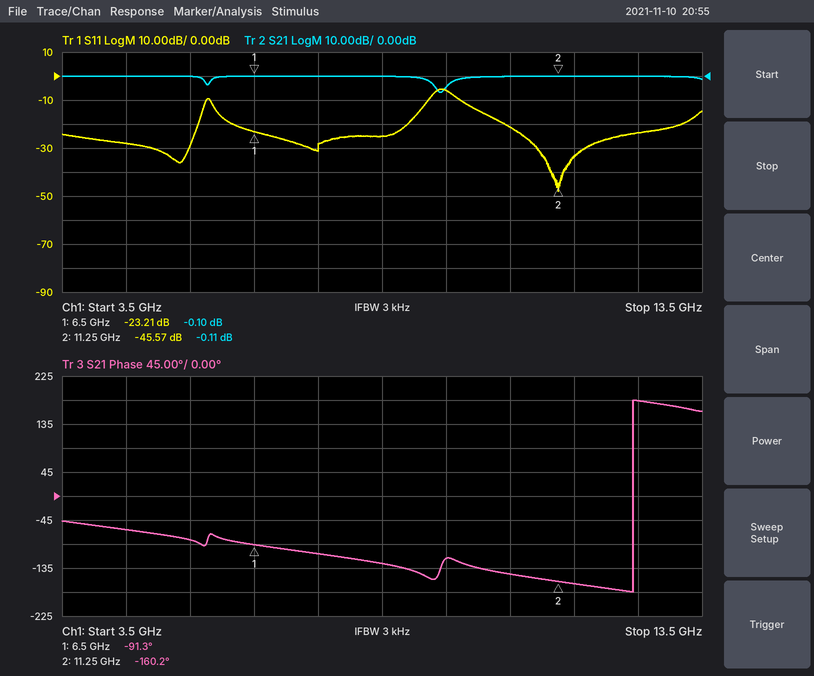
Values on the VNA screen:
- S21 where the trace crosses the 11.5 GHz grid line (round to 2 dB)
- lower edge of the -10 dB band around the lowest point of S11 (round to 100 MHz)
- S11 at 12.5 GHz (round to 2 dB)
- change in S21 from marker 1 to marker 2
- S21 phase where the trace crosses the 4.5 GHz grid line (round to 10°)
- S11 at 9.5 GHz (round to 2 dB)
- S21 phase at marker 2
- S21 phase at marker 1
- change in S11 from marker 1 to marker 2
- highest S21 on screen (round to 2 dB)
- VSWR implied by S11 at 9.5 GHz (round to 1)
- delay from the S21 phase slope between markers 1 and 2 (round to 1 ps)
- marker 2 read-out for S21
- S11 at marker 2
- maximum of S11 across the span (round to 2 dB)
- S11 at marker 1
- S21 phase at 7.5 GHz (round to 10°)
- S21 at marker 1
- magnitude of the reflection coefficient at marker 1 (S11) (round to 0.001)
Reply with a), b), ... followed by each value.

a) 0 dB
b) 9.7 GHz
c) -24 dB
d) -0.01 dB
e) -60°
f) -6 dB
g) -160.2°
h) -91.3°
i) -22.36 dB
j) 0 dB
k) 3
l) 40 ps
m) -0.11 dB
n) -45.57 dB
o) -6 dB
p) -23.21 dB
q) -110°
r) -0.10 dB
s) 0.069
